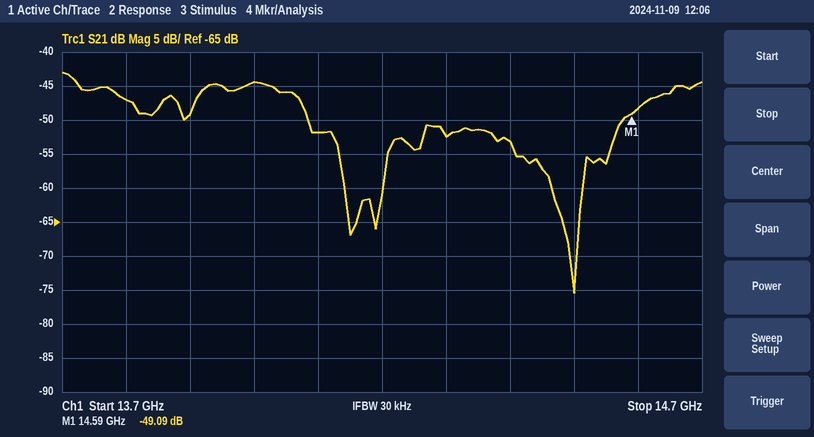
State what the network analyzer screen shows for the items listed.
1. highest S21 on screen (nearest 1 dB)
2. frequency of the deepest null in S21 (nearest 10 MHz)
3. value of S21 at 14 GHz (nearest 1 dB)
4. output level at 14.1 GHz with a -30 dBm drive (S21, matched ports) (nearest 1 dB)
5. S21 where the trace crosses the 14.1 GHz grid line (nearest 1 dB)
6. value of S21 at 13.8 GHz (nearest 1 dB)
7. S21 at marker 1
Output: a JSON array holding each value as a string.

["-43 dB", "14.50 GHz", "-44 dB", "-82 dBm", "-52 dB", "-47 dB", "-49.09 dB"]
